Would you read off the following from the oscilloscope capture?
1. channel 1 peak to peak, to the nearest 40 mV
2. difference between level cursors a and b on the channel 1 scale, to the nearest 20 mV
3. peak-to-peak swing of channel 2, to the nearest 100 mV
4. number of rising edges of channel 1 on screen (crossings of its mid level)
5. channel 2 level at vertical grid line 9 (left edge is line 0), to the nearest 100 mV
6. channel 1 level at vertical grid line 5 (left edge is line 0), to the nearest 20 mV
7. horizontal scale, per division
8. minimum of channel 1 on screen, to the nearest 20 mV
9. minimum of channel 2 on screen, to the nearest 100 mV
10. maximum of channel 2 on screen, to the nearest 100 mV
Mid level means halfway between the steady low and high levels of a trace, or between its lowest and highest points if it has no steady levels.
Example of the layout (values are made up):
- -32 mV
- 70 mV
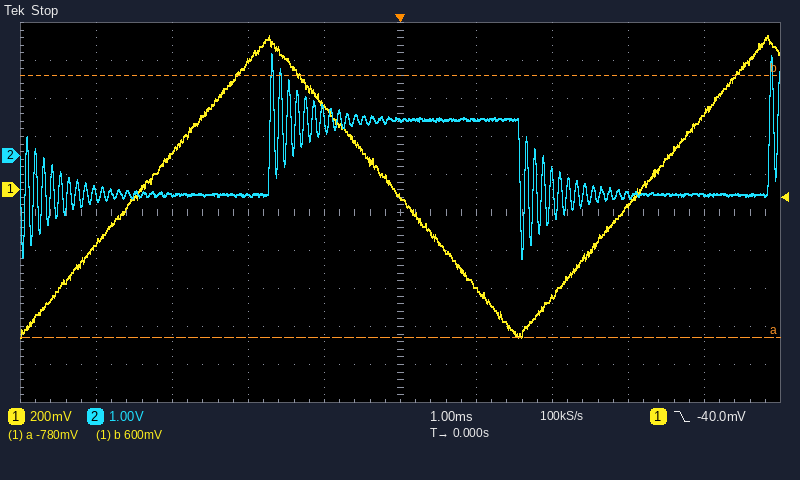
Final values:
- 1.60 V
- 1.38 V
- 5.4 V
- 2
- -1.0 V
- -40 mV
- 1 ms
- -780 mV
- -2.7 V
- 2.7 V
